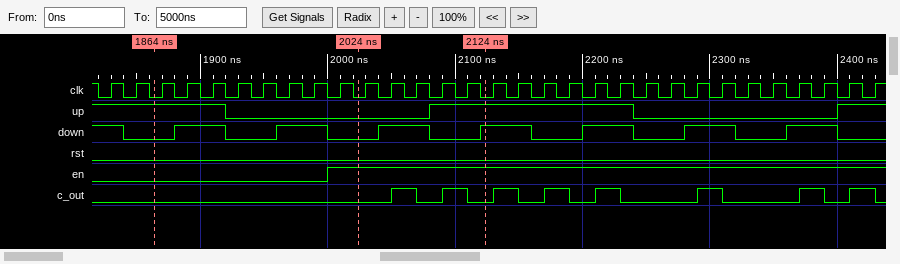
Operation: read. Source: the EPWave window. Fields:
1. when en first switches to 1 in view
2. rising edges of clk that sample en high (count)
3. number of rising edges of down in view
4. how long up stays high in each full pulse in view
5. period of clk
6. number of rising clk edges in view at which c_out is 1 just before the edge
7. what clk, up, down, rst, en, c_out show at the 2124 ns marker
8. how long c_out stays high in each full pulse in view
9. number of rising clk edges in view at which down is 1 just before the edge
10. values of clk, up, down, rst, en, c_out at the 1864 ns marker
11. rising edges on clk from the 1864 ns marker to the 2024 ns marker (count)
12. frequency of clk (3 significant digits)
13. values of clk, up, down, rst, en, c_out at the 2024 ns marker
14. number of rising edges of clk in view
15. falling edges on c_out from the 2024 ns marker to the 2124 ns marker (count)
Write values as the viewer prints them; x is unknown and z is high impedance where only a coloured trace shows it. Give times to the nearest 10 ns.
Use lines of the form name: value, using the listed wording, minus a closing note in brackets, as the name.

when en first switches to 1 in view: 2000 ns
rising edges of clk that sample en high: 22
number of rising edges of down in view: 7
how long up stays high in each full pulse in view: 160 ns
period of clk: 20 ns
number of rising clk edges in view at which c_out is 1 just before the edge: 8
what clk, up, down, rst, en, c_out show at the 2124 ns marker: clk=0, up=1, down=1, rst=0, en=1, c_out=0
how long c_out stays high in each full pulse in view: 20 ns, 20 ns, 20 ns, 20 ns, 20 ns, 20 ns, 20 ns, 20 ns
number of rising clk edges in view at which down is 1 just before the edge: 15
values of clk, up, down, rst, en, c_out at the 1864 ns marker: clk=0, up=1, down=0, rst=0, en=0, c_out=0
rising edges on clk from the 1864 ns marker to the 2024 ns marker: 8
frequency of clk: 50.0 MHz
values of clk, up, down, rst, en, c_out at the 2024 ns marker: clk=0, up=0, down=0, rst=0, en=1, c_out=0
number of rising edges of clk in view: 31
falling edges on c_out from the 2024 ns marker to the 2124 ns marker: 2
